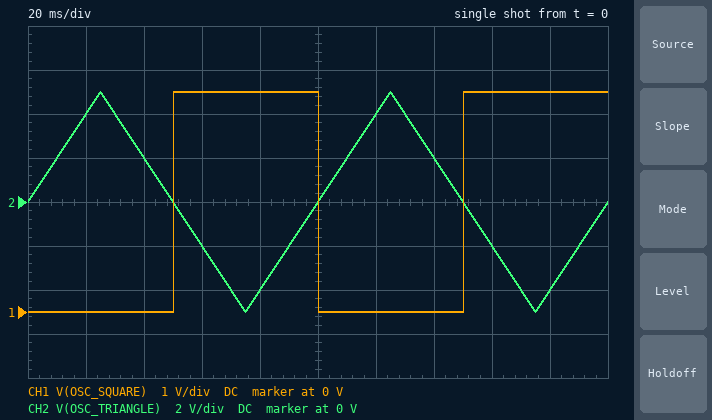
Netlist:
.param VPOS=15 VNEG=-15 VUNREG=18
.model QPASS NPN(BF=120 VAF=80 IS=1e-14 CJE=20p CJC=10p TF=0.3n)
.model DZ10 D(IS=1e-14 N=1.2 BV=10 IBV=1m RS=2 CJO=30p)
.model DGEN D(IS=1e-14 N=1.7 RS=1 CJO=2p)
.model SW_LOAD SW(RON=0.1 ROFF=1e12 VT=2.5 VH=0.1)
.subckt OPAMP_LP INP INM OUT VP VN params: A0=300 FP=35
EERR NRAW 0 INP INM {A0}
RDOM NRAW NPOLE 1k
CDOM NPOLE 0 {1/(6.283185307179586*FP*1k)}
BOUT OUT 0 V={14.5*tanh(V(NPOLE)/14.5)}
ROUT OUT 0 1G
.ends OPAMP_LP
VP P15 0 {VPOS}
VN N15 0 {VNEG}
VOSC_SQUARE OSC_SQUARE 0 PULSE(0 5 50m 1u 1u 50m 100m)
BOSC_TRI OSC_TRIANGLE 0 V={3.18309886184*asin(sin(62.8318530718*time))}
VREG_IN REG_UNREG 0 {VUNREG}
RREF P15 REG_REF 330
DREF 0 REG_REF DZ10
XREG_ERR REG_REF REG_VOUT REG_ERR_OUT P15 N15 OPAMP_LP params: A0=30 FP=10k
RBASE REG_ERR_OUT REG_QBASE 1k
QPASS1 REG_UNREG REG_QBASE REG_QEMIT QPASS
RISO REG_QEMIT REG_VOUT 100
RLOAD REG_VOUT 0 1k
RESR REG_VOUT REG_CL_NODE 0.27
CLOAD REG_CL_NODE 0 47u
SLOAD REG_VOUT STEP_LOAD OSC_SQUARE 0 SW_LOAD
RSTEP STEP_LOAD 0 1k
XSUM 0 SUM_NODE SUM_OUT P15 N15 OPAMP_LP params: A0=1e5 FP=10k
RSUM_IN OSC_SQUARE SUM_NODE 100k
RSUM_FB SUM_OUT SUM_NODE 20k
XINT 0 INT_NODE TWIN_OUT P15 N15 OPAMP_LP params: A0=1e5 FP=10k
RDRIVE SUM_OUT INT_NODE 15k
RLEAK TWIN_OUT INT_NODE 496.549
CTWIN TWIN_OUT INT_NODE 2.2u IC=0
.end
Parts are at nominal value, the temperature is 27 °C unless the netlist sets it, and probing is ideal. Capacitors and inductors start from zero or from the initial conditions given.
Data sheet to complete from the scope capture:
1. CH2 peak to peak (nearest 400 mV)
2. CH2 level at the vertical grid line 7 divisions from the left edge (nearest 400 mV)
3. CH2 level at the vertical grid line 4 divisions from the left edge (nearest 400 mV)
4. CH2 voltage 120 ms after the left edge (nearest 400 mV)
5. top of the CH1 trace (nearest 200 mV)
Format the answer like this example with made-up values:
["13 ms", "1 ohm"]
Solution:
["10.0 V", "2.0 V", "-4.0 V", "4.0 V", "5.0 V"]
